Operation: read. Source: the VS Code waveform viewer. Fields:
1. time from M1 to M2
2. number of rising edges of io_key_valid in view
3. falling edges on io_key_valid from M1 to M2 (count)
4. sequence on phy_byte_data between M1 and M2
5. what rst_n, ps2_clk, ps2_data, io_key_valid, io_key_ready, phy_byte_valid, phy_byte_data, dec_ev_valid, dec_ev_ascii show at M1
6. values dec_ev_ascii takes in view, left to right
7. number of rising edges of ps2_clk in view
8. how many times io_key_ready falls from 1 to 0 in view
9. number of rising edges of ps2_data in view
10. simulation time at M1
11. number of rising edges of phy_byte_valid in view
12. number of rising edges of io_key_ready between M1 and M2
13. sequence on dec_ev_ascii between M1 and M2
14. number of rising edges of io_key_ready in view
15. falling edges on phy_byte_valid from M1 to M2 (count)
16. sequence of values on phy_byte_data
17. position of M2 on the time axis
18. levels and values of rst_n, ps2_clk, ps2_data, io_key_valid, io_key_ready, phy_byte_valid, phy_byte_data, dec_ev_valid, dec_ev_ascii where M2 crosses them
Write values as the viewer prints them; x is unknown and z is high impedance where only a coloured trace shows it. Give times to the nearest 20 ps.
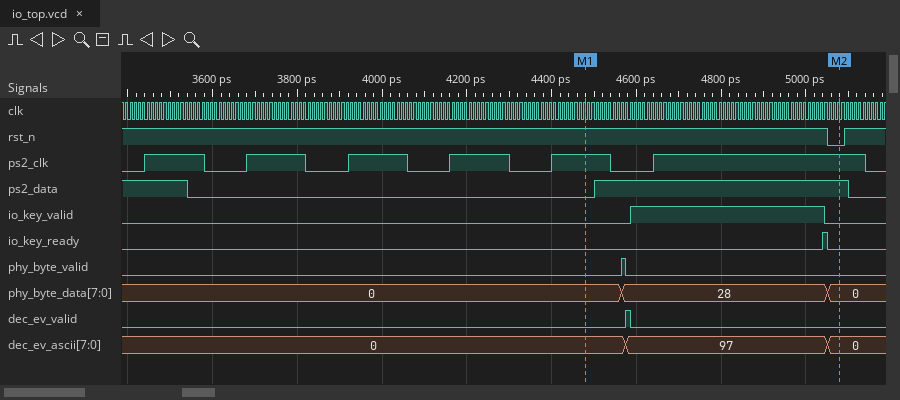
600 ps
1
1
0, 28, 0
rst_n=1, ps2_clk=1, ps2_data=0, io_key_valid=0, io_key_ready=0, phy_byte_valid=0, phy_byte_data=0, dec_ev_valid=0, dec_ev_ascii=0
0, 97, 0
6
1
1
4480 ps
1
1
0, 97, 0
1
1
0, 28, 0
5080 ps
rst_n=0, ps2_clk=1, ps2_data=1, io_key_valid=0, io_key_ready=0, phy_byte_valid=0, phy_byte_data=0, dec_ev_valid=0, dec_ev_ascii=0
